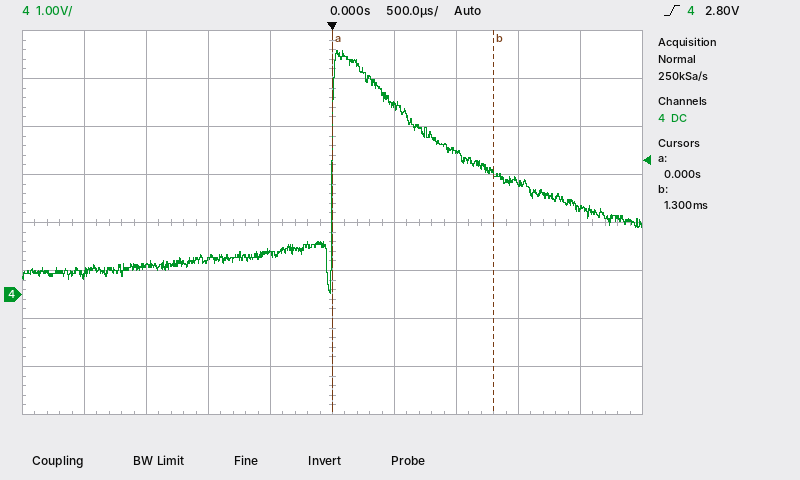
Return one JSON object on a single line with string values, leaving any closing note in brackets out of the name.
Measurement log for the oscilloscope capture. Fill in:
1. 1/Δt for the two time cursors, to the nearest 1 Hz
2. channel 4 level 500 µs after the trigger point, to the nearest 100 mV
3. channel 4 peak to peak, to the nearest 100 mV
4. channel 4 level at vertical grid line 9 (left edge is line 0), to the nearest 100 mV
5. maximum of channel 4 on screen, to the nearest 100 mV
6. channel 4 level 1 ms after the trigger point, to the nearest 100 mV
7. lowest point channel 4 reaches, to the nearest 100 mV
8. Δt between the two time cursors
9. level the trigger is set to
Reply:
{"1/Δt for the two time cursors, to the nearest 1 Hz": "769 Hz", "channel 4 level 500 µs after the trigger point, to the nearest 100 mV": "3.9 V", "channel 4 peak to peak, to the nearest 100 mV": "5.1 V", "channel 4 level at vertical grid line 9 (left edge is line 0), to the nearest 100 mV": "1.8 V", "maximum of channel 4 on screen, to the nearest 100 mV": "5.1 V", "channel 4 level 1 ms after the trigger point, to the nearest 100 mV": "3.0 V", "lowest point channel 4 reaches, to the nearest 100 mV": "0.0 V", "Δt between the two time cursors": "1.30 ms", "level the trigger is set to": "2.80 V"}
